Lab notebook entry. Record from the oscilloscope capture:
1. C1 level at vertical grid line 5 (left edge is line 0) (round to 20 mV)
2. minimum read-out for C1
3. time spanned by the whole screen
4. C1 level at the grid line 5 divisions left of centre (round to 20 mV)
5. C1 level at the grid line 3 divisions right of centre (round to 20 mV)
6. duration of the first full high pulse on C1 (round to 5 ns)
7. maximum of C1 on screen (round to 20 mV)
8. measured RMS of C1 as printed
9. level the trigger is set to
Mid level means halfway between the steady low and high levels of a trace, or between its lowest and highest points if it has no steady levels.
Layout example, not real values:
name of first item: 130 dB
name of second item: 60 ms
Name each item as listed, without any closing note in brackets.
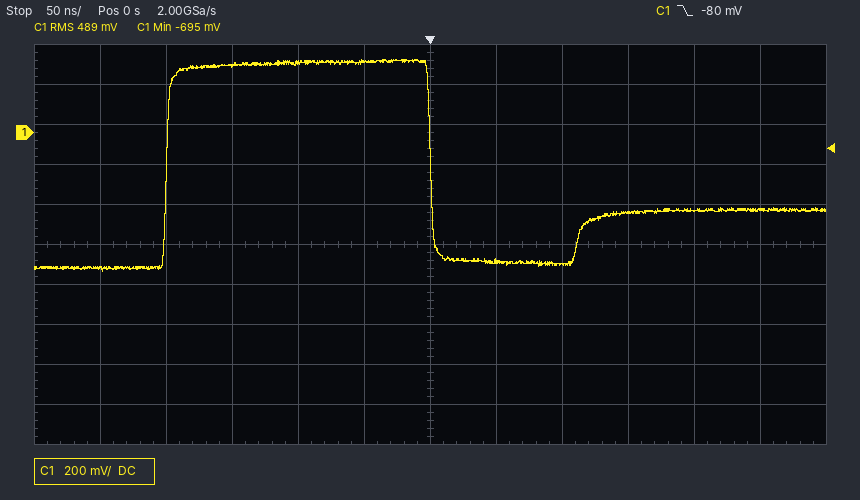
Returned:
C1 level at vertical grid line 5 (left edge is line 0): 360 mV
minimum read-out for C1: -695 mV
time spanned by the whole screen: 600 ns
C1 level at the grid line 5 divisions left of centre: -680 mV
C1 level at the grid line 3 divisions right of centre: -400 mV
duration of the first full high pulse on C1: 200 ns
maximum of C1 on screen: 360 mV
measured RMS of C1 as printed: 489 mV
level the trigger is set to: -80 mV
